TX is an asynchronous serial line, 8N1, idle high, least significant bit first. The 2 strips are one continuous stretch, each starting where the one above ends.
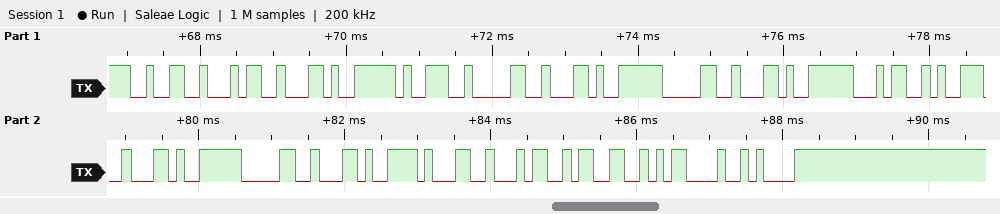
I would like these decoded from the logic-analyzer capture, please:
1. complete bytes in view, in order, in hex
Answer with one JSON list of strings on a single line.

["0x32 0x34 0x2C 0x39 0x30 0x2C 0x30 0x2C 0x34 0x39 0x2C 0x30 0x2C 0x31 0x34 0x33 0x0D 0x0A"]
